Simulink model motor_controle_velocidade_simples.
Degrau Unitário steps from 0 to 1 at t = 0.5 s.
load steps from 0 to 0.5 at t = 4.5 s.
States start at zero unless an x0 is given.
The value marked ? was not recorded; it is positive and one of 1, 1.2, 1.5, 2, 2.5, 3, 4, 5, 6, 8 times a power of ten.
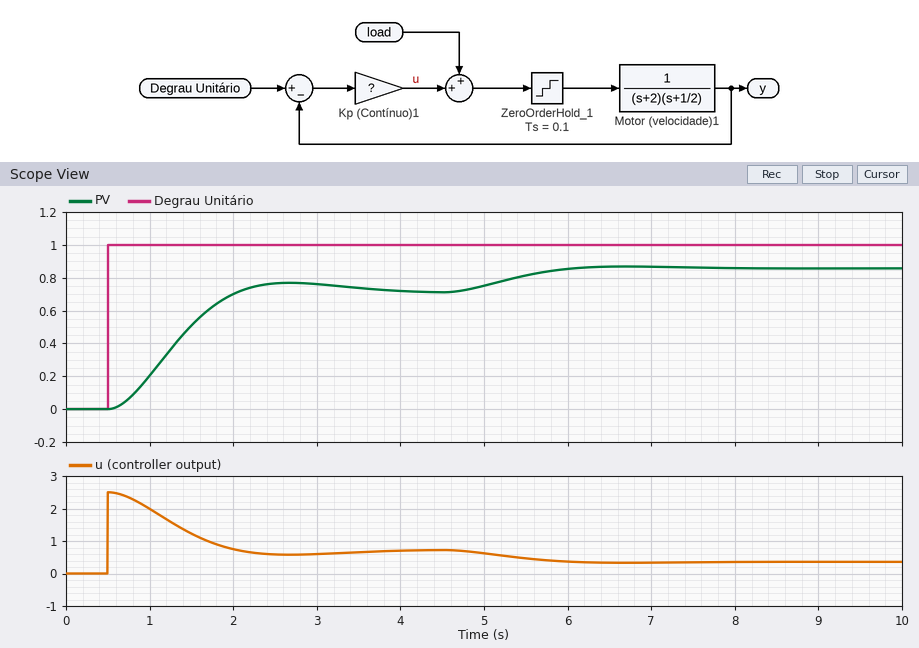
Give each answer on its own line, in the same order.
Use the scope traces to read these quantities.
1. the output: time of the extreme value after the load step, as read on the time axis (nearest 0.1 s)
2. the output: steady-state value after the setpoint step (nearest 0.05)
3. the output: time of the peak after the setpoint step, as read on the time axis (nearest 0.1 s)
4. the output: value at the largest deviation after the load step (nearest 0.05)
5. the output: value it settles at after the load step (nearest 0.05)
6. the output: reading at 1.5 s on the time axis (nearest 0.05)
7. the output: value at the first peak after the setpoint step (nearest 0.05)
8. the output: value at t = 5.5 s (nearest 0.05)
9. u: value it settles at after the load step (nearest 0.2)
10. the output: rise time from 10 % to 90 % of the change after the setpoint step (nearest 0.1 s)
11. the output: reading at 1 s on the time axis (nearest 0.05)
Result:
6.7 s
0.70
2.7 s
0.85
0.85
0.50
0.75
0.80
0.4
1.0 s
0.20
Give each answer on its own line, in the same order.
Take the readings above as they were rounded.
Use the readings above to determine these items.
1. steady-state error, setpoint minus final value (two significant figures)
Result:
0.30
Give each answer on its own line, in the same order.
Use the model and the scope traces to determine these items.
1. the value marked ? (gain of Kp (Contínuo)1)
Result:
2.5
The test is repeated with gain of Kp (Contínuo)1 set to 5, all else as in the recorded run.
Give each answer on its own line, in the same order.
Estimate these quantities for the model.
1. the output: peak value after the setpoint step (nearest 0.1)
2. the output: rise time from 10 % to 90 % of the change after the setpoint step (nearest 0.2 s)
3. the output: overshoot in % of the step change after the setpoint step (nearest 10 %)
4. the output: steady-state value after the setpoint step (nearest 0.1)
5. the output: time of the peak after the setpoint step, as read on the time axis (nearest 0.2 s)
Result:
1.0
0.6 s
20 %
0.8
2.0 s
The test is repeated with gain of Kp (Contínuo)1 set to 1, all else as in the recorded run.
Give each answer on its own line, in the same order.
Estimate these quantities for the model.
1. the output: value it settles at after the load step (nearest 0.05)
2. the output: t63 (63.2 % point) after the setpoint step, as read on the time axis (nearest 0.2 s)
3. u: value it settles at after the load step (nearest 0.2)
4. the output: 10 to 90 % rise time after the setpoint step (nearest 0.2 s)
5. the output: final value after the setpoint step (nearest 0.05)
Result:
0.75
1.8 s
0.2
2.0 s
0.50
